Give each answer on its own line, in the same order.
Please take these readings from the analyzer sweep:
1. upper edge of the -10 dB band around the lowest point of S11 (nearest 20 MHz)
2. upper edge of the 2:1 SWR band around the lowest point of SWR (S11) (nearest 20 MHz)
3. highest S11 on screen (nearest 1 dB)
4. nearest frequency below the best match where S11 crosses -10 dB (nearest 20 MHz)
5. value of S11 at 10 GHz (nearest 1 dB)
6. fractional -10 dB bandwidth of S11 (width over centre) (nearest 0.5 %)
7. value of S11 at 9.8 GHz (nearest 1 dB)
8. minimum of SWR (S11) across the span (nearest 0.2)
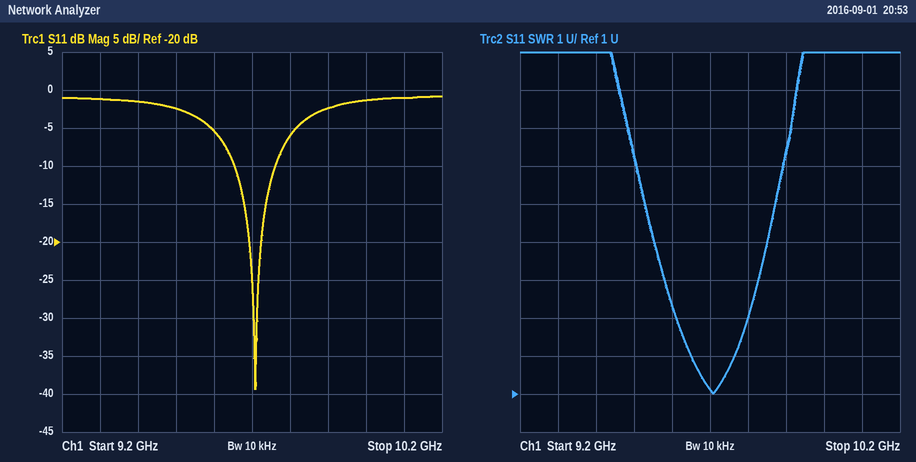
9.76 GHz
9.76 GHz
-1 dB
9.66 GHz
-1 dB
1.0 %
-6 dB
1.0
